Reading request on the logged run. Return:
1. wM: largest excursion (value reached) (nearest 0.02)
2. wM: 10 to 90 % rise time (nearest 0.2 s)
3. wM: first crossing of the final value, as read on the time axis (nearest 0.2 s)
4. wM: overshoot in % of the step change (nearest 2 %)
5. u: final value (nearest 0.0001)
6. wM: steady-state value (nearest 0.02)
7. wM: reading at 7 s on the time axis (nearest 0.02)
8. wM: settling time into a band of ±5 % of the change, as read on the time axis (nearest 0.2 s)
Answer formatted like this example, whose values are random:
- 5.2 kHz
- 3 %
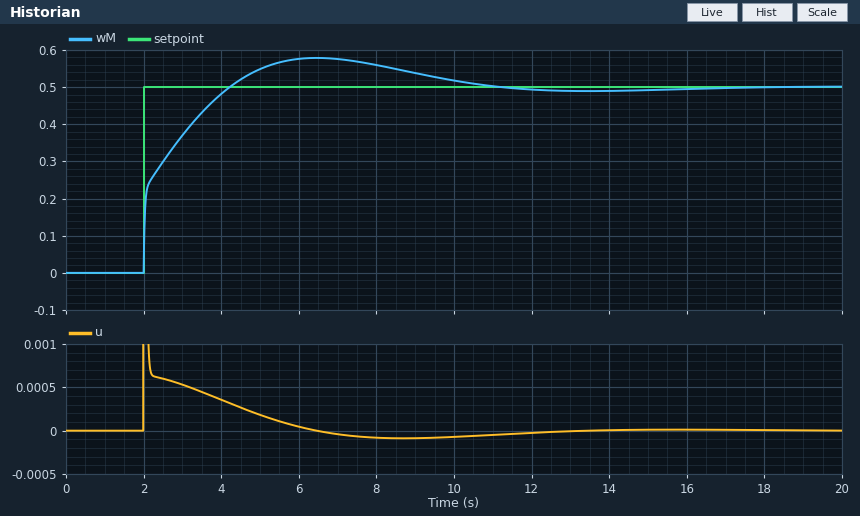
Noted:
- 0.58
- 1.6 s
- 4.2 s
- 16 %
- 0.0000
- 0.50
- 0.58
- 9.6 s
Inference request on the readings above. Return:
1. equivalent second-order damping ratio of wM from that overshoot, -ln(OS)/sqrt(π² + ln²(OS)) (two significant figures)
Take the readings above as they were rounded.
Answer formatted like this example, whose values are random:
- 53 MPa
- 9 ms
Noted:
- 0.50
